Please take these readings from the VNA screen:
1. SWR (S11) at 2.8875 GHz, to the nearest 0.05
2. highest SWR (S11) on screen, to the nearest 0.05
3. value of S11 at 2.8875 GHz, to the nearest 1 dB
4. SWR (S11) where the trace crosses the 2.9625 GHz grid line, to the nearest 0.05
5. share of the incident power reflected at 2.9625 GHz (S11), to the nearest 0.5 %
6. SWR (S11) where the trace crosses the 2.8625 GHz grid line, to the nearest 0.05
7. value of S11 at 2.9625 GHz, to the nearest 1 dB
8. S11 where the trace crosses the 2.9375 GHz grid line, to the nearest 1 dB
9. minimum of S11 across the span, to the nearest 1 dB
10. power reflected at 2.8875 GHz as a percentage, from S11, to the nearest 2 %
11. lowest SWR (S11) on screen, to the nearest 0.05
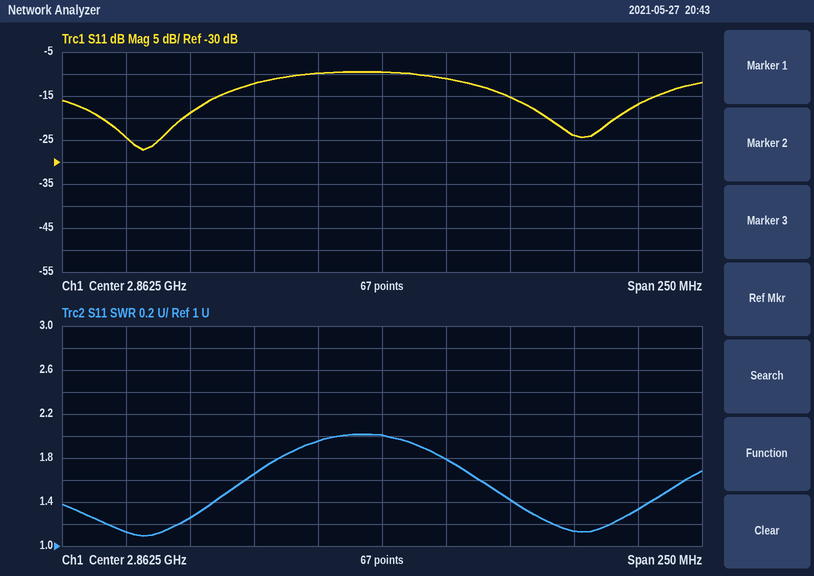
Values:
1.80
2.00
-11 dB
1.35
2.0 %
2.00
-17 dB
-24 dB
-27 dB
8 %
1.10
